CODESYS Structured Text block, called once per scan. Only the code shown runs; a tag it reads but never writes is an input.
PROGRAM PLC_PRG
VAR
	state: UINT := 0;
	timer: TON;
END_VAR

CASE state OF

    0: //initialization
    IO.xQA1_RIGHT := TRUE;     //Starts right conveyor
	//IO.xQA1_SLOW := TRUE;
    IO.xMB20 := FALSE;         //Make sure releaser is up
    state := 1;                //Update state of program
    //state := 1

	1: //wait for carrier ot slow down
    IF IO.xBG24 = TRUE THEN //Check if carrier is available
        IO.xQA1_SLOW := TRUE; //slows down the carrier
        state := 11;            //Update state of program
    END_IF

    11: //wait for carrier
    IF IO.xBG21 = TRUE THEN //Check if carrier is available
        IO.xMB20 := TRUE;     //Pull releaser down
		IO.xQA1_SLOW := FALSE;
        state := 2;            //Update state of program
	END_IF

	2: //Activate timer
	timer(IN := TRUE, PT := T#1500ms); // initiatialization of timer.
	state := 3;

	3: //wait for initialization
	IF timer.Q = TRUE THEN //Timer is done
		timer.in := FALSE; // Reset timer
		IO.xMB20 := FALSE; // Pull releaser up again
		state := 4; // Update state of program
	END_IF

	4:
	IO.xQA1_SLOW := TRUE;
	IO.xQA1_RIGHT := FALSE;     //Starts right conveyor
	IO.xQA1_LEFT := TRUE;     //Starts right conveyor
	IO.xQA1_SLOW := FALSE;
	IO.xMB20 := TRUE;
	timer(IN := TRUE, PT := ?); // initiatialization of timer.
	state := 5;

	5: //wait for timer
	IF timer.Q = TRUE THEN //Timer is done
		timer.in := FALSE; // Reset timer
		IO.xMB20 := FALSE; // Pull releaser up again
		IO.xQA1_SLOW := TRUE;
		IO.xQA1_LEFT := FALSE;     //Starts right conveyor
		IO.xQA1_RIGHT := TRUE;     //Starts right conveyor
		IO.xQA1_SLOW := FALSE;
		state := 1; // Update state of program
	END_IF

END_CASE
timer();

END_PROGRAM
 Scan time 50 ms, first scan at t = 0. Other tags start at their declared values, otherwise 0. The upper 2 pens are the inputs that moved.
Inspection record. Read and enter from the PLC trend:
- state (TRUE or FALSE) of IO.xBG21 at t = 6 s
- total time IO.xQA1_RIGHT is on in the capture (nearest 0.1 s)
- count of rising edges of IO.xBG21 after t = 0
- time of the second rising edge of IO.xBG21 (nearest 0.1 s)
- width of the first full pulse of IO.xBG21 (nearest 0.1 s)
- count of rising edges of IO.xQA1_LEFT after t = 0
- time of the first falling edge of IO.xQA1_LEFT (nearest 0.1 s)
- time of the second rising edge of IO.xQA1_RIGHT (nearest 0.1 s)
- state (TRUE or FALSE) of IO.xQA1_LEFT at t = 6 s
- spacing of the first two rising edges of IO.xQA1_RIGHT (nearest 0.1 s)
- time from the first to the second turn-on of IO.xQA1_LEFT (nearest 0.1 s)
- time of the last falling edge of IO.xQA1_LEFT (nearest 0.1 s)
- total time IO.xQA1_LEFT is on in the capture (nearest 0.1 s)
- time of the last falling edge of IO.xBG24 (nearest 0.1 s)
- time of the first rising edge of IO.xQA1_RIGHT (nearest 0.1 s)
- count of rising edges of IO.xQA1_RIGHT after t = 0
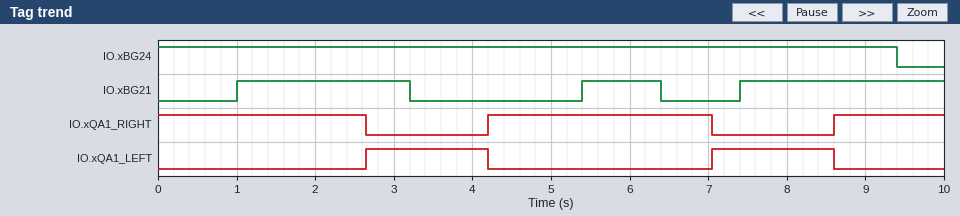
TRUE
6.9 s
3
5.4 s
2.2 s
2
4.2 s
8.6 s
FALSE
4.4 s
4.4 s
8.6 s
3.1 s
9.4 s
4.2 s
2
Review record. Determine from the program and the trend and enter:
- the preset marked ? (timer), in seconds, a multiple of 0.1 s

1.5 s
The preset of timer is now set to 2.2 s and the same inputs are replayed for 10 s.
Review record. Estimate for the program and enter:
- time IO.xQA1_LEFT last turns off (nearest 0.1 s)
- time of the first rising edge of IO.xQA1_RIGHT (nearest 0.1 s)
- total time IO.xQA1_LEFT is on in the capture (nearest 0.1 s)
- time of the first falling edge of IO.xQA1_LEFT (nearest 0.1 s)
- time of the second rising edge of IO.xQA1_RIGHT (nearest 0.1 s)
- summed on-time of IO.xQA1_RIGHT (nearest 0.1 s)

9.3 s
4.9 s
4.5 s
4.9 s
9.3 s
5.5 s
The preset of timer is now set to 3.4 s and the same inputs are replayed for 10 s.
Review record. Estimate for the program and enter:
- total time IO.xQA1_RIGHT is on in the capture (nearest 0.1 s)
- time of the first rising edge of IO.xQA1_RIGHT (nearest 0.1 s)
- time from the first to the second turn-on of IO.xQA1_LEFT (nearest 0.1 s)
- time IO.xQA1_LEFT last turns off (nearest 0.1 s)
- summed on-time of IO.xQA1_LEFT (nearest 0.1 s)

4.4 s
6.1 s
5.2 s
6.1 s
5.6 s
